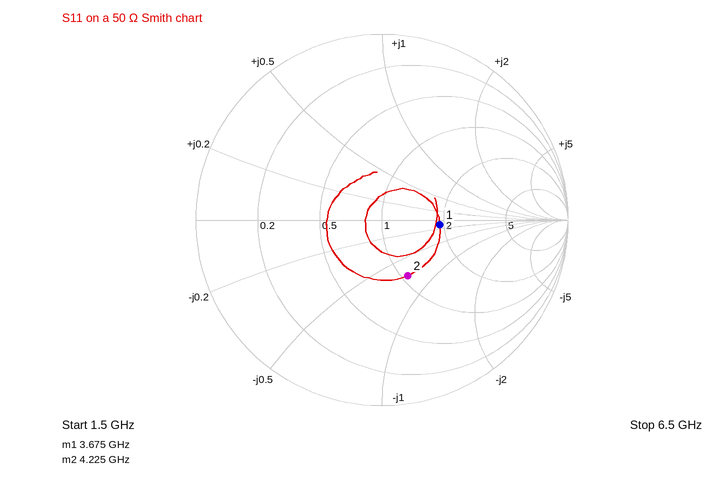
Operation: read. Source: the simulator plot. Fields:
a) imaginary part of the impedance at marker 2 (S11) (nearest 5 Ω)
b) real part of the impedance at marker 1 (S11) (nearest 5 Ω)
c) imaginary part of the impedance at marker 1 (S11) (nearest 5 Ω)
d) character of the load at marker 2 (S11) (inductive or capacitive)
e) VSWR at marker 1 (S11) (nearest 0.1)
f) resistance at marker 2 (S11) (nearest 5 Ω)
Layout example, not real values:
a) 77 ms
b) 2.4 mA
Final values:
a) -35 Ω
b) 95 Ω
c) -5 Ω
d) capacitive
e) 1.9
f) 55 Ω
